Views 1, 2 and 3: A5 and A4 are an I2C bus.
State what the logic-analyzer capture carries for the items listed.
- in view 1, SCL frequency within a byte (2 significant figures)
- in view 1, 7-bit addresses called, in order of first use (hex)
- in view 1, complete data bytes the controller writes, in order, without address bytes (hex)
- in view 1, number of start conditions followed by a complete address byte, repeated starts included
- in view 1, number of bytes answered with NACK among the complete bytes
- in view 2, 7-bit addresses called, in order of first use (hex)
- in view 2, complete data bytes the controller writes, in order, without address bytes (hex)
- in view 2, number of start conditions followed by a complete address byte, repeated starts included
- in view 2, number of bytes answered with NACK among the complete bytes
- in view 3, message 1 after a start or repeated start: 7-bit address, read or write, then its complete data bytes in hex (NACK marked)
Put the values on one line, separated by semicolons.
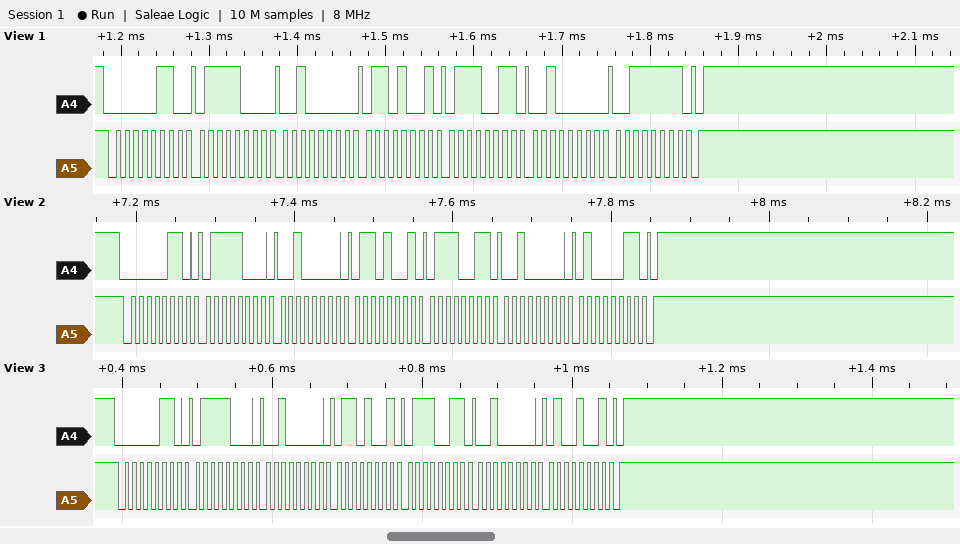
100 kHz; 0x03; 78 20 69 73 20 3F; 1; 0; 0x03; 78 20 69 73 20 43; 1; 0; 0x03 write: 78 20 69 73 20 49
